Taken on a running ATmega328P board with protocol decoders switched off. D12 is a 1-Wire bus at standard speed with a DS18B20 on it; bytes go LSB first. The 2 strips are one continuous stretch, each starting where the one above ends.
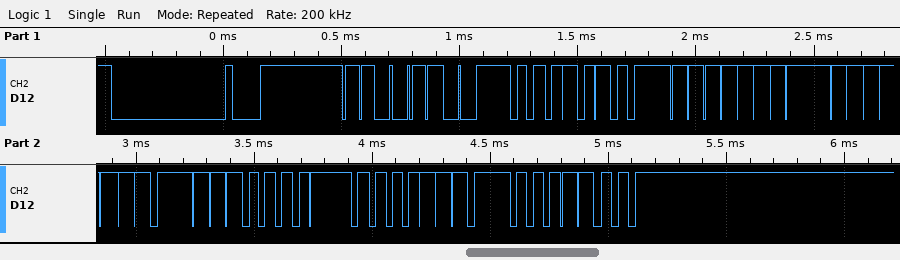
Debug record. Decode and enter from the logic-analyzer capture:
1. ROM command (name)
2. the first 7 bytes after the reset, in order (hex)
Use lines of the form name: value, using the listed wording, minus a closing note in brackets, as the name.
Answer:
ROM command: Read ROM
the first 7 bytes after the reset, in order: 33 28 FF 7F 87 70 18
